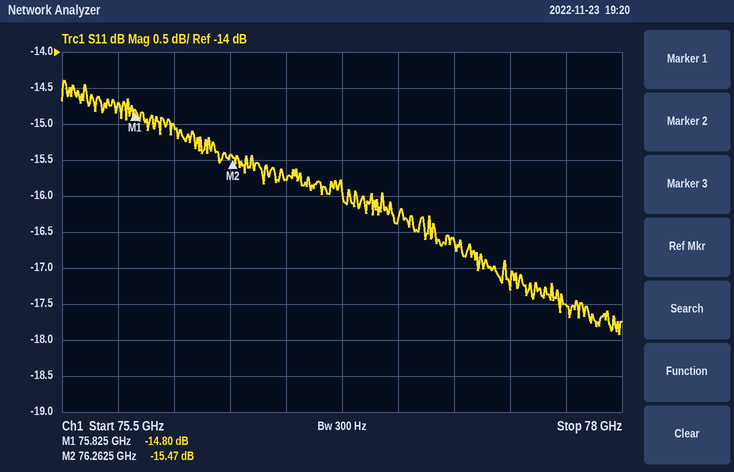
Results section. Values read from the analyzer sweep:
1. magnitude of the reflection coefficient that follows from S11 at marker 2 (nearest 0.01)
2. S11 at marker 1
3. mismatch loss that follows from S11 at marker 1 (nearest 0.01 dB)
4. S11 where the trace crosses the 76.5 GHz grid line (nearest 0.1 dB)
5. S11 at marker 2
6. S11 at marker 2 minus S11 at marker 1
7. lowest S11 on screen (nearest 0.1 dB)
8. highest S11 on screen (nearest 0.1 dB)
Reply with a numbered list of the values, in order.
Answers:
1. 0.17
2. -14.80 dB
3. 0.15 dB
4. -15.8 dB
5. -15.47 dB
6. -0.67 dB
7. -17.9 dB
8. -14.4 dB
